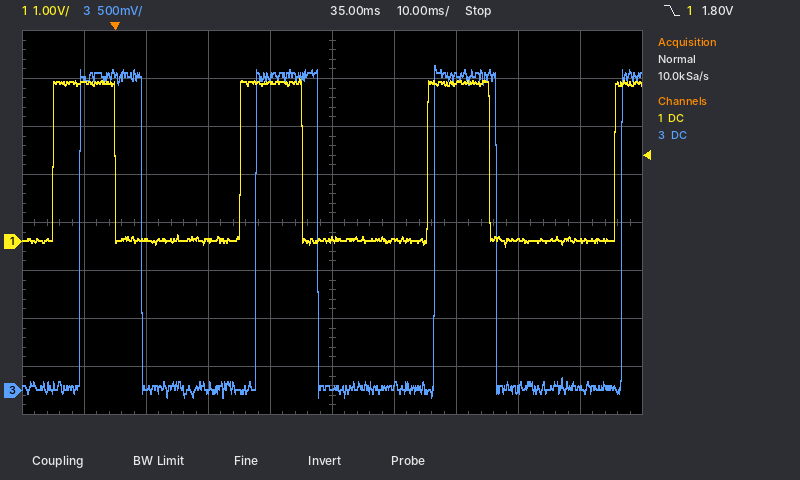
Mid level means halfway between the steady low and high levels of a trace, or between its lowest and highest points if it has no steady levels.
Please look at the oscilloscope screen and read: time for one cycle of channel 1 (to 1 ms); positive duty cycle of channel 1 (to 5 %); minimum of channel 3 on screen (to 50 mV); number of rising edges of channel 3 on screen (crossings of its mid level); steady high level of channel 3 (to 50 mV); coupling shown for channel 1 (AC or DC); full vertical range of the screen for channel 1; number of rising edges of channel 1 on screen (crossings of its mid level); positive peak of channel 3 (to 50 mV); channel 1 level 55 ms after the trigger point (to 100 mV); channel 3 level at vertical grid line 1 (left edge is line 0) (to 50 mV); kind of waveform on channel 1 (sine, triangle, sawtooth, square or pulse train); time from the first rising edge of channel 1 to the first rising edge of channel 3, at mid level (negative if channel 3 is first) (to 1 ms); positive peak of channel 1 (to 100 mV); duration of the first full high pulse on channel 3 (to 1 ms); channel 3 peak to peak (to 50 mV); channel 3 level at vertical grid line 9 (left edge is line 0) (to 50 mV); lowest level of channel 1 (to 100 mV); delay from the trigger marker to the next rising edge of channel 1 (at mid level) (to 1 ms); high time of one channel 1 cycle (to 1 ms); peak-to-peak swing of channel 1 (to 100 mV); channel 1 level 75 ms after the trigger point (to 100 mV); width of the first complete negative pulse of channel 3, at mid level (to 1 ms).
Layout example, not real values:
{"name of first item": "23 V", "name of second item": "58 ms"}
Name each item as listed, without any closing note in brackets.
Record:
{"time for one cycle of channel 1": "30 ms", "positive duty cycle of channel 1": "35 %", "minimum of channel 3 on screen": "-50 mV", "number of rising edges of channel 3 on screen": "4", "steady high level of channel 3": "3.30 V", "coupling shown for channel 1": "DC", "full vertical range of the screen for channel 1": "8 V", "number of rising edges of channel 1 on screen": "4", "positive peak of channel 3": "3.40 V", "channel 1 level 55 ms after the trigger point": "3.3 V", "channel 3 level at vertical grid line 1 (left edge is line 0)": "3.25 V", "kind of waveform on channel 1": "pulse train", "time from the first rising edge of channel 1 to the first rising edge of channel 3, at mid level (negative if channel 3 is first)": "+4 ms", "positive peak of channel 1": "3.4 V", "duration of the first full high pulse on channel 3": "10 ms", "channel 3 peak to peak": "3.45 V", "channel 3 level at vertical grid line 9 (left edge is line 0)": "50 mV", "lowest level of channel 1": "-100 mV", "delay from the trigger marker to the next rising edge of channel 1 (at mid level)": "20 ms", "high time of one channel 1 cycle": "10 ms", "peak-to-peak swing of channel 1": "3.5 V", "channel 1 level 75 ms after the trigger point": "0.0 V", "width of the first complete negative pulse of channel 3, at mid level": "18 ms"}
